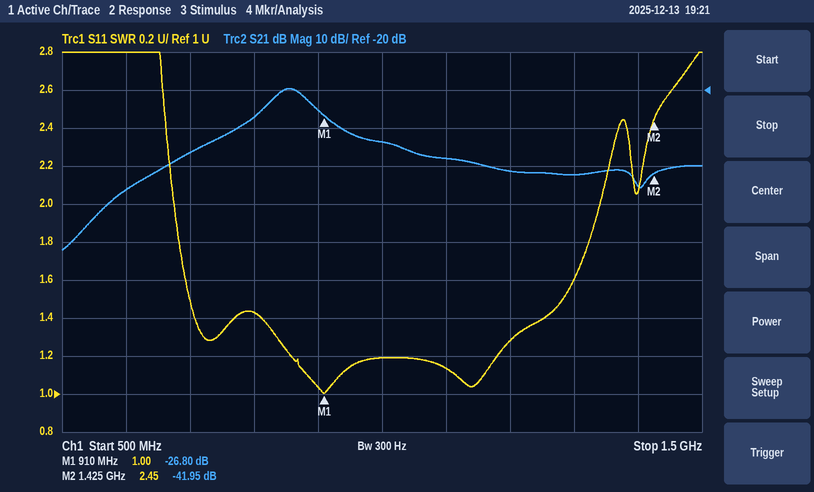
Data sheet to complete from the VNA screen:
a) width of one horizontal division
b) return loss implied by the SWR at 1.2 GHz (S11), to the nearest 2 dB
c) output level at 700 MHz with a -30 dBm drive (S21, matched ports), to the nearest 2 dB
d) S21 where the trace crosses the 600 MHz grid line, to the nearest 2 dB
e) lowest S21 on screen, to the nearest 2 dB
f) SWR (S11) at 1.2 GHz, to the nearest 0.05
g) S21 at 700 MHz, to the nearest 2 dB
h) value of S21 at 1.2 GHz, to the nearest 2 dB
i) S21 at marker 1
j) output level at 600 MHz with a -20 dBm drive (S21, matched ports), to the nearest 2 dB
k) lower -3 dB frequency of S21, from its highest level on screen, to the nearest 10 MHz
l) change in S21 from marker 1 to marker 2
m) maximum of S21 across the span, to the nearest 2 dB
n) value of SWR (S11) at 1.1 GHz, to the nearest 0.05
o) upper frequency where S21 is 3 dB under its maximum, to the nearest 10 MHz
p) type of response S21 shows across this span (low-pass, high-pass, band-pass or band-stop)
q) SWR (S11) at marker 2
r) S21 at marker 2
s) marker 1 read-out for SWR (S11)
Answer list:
100 MHz
18 dB
-66 dBm
-46 dB
-62 dB
1.30
-36 dB
-42 dB
-26.80 dB
-66 dBm
830 MHz
-15.15 dB
-20 dB
1.15
880 MHz
band-pass
2.45
-41.95 dB
1.00
